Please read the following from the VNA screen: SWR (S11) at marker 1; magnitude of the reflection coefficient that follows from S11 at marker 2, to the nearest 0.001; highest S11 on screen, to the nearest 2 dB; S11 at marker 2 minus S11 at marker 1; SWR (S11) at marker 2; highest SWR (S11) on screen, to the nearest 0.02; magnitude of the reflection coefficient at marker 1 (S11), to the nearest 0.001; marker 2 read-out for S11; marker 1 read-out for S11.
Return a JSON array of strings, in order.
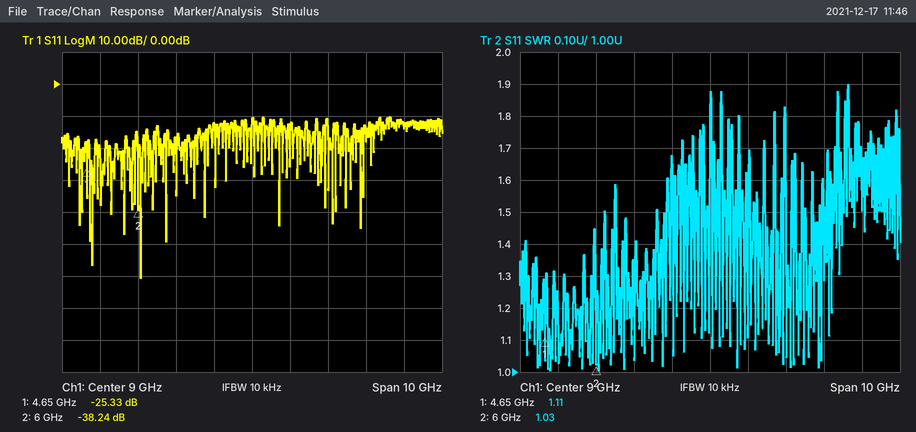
["1.11", "0.012", "-10 dB", "-12.91 dB", "1.03", "1.90", "0.054", "-38.24 dB", "-25.33 dB"]
